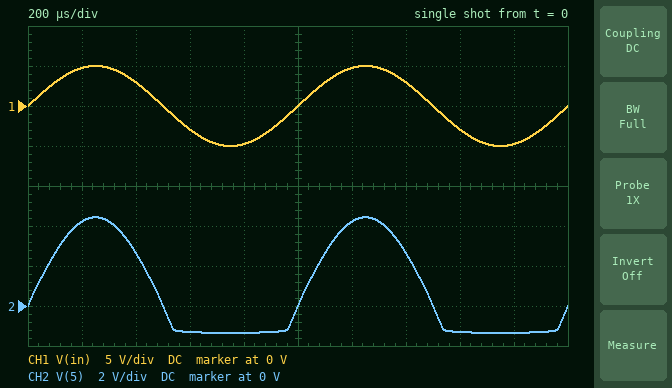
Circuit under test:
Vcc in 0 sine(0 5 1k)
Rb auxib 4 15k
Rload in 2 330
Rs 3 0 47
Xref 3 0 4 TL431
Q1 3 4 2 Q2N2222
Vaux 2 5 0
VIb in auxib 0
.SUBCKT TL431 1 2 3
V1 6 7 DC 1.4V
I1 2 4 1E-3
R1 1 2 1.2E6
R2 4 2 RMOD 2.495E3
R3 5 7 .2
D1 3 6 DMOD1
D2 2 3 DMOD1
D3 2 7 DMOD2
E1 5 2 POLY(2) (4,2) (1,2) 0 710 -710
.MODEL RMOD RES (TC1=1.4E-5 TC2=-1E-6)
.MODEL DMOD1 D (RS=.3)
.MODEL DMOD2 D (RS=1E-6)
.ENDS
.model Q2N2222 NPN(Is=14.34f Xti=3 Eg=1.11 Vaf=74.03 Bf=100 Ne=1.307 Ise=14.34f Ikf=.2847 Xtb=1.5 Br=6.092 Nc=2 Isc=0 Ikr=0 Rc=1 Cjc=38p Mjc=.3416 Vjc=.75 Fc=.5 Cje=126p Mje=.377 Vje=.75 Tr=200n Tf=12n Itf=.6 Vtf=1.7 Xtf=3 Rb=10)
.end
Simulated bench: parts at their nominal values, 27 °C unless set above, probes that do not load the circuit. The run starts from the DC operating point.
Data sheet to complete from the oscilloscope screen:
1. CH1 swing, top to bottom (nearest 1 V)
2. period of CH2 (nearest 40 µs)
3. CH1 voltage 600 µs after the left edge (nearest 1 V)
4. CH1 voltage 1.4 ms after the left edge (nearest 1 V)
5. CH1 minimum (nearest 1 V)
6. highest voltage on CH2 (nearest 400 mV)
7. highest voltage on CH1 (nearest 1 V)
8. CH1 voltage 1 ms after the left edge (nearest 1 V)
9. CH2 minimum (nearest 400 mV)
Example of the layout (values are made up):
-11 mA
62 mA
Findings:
10 V
1.00 ms
-3 V
3 V
-5 V
4.4 V
5 V
0 V
-1.2 V
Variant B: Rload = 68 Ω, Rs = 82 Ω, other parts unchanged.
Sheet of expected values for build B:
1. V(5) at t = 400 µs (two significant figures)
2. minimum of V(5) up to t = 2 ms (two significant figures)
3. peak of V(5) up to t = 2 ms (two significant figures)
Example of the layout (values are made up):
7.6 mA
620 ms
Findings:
2.9 V
-1.8 V
4.9 V
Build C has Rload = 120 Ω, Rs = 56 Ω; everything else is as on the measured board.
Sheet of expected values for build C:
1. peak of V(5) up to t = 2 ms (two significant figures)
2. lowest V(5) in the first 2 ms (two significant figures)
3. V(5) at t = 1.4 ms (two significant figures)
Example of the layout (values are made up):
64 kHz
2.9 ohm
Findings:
4.8 V
-1.5 V
2.8 V
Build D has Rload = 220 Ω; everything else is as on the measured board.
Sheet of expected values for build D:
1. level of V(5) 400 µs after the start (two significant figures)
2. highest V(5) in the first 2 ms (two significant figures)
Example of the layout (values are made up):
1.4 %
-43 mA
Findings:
2.7 V
4.6 V
